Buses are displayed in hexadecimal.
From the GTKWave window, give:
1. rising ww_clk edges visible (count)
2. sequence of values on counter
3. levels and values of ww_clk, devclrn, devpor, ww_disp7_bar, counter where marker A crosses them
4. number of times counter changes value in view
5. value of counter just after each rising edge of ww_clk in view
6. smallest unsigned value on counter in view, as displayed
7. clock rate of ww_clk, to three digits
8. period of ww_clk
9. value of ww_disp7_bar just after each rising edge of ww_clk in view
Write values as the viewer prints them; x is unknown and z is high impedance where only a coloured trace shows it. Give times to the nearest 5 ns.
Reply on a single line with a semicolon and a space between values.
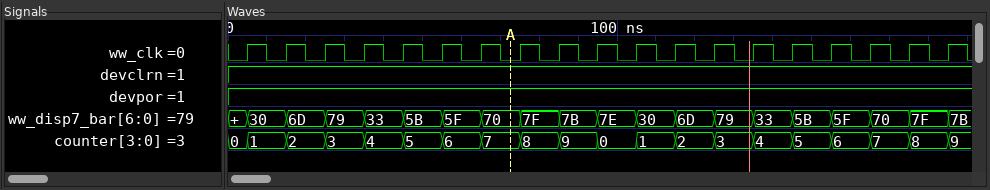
19; 0, 1, 2, 3, 4, 5, 6, 7, 8, 9, 0, 1, 2, 3, 4, 5, 6, 7, 8, 9; ww_clk=0, devclrn=1, devpor=1, ww_disp7_bar=70, counter=7; 19; 1, 2, 3, 4, 5, 6, 7, 8, 9, 0, 1, 2, 3, 4, 5, 6, 7, 8, 9; 0; 100 MHz; 10 ns; 30, 6D, 79, 33, 5B, 5F, 70, 7F, 7B, 7E, 30, 6D, 79, 33, 5B, 5F, 70, 7F, 7B
